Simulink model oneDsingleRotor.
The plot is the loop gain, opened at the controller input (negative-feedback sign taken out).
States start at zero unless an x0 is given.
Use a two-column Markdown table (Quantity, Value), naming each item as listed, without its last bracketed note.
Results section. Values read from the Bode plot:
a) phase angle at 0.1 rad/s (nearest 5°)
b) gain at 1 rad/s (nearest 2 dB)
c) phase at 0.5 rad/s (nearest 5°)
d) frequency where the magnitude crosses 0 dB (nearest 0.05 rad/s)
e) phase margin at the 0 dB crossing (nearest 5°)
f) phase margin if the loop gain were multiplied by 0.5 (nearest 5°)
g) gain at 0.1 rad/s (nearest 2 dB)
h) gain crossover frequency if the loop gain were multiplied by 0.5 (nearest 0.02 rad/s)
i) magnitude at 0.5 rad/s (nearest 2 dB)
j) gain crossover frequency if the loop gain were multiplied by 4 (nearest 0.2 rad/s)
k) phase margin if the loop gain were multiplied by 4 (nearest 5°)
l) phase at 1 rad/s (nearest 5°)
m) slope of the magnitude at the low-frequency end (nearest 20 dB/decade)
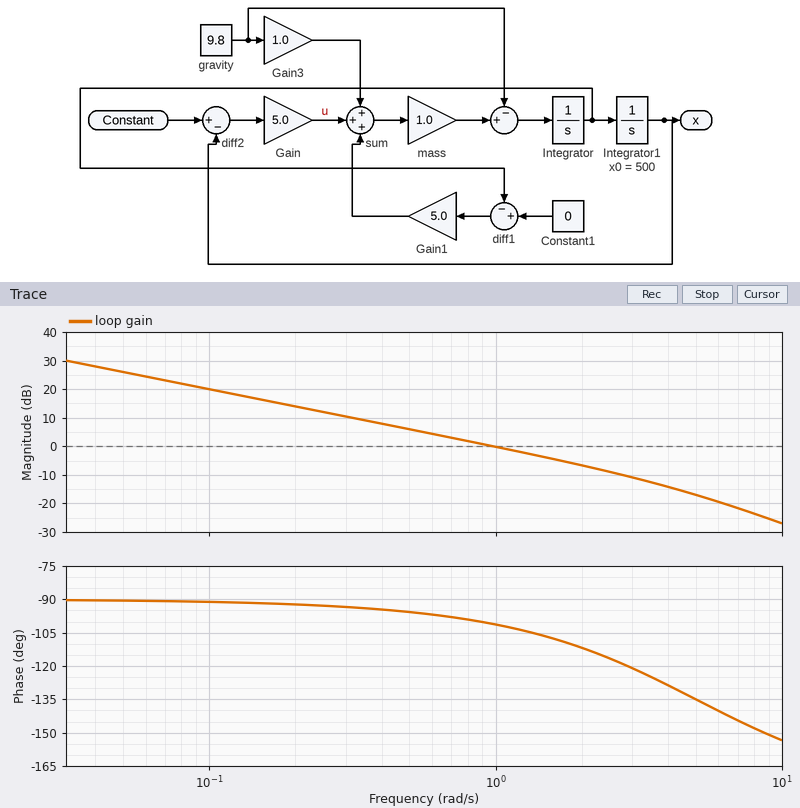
| Quantity | Value |
|---|---|
| phase angle at 0.1 rad/s | -90° |
| gain at 1 rad/s | 0 dB |
| phase at 0.5 rad/s | -95° |
| frequency where the magnitude crosses 0 dB | 1.00 rad/s |
| phase margin at the 0 dB crossing | 80° |
| phase margin if the loop gain were multiplied by 0.5 | 85° |
| gain at 0.1 rad/s | 20 dB |
| gain crossover frequency if the loop gain were multiplied by 0.5 | 0.50 rad/s |
| magnitude at 0.5 rad/s | 6 dB |
| gain crossover frequency if the loop gain were multiplied by 4 | 3.4 rad/s |
| phase margin if the loop gain were multiplied by 4 | 55° |
| phase at 1 rad/s | -100° |
| slope of the magnitude at the low-frequency end | -20 dB/decade |
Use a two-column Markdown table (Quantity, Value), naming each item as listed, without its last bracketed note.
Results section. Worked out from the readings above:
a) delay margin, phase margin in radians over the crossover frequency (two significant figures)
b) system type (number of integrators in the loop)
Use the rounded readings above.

| Quantity | Value |
|---|---|
| delay margin, phase margin in radians over the crossover frequency | 1.4 s |
| system type | 1 |
